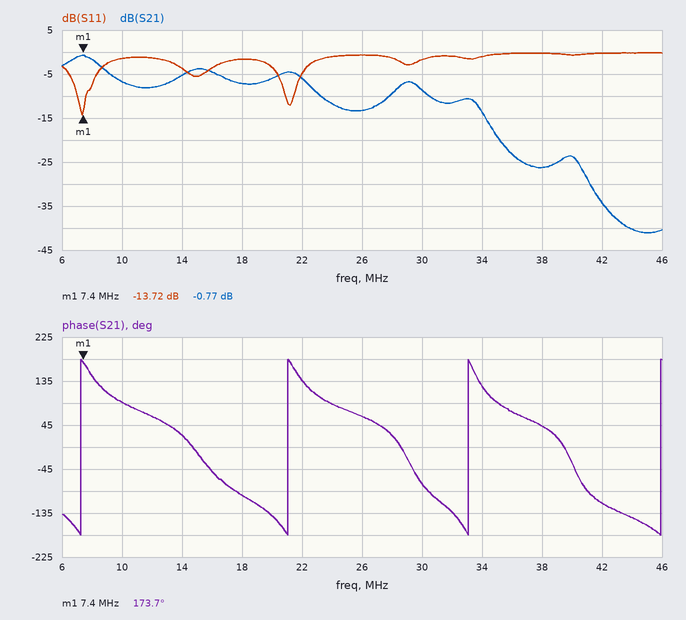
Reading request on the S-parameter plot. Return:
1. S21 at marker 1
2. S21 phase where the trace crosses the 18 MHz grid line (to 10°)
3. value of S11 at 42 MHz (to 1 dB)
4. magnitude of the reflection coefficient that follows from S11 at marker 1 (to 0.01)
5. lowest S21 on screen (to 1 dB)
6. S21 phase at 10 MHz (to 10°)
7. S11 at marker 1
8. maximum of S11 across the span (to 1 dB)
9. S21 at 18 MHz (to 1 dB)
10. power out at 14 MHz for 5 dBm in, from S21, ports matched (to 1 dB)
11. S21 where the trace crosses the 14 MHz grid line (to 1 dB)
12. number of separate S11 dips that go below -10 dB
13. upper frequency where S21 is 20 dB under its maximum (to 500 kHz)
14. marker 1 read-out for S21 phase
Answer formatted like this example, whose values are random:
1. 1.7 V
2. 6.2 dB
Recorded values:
1. -0.77 dB
2. -100°
3. 0 dB
4. 0.21
5. -41 dB
6. 90°
7. -13.72 dB
8. 0 dB
9. -7 dB
10. 0 dBm
11. -5 dB
12. 2
13. 35.5 MHz
14. 173.7°
